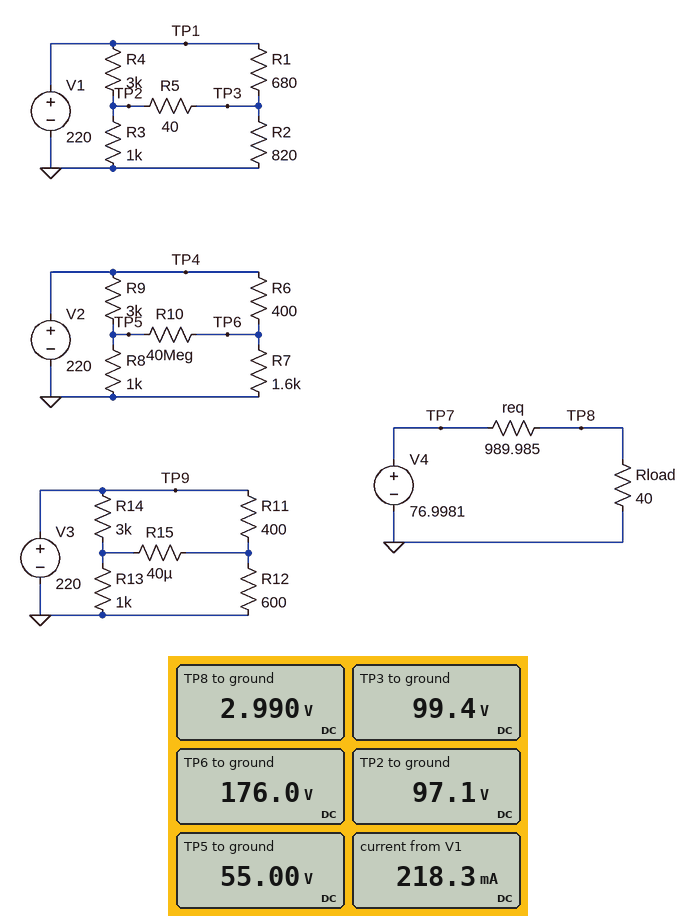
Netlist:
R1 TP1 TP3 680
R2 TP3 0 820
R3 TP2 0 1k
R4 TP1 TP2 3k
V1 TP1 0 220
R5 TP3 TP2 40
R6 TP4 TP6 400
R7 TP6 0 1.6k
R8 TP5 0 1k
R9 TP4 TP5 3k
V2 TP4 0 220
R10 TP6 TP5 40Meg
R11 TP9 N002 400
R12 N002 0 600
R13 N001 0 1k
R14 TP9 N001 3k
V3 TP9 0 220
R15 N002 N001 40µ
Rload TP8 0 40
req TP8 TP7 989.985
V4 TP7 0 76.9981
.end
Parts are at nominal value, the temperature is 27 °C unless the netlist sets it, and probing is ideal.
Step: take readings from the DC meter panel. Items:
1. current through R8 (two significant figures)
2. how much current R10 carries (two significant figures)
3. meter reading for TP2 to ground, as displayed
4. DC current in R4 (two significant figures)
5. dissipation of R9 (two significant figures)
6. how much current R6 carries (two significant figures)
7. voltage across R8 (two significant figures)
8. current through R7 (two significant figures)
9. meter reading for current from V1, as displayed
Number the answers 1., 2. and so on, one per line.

1. 55 mA
2. 3.0 µA
3. 97.1 V
4. 41 mA
5. 9.1 W
6. 110 mA
7. 55 V
8. 110 mA
9. 218.3 mA
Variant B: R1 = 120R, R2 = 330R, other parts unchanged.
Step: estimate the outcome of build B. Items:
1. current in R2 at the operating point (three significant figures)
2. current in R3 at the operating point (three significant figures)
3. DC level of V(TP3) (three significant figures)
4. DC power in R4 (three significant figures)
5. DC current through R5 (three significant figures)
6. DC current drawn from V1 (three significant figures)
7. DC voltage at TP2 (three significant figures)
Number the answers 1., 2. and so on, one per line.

1. 457 mA
2. 146 mA
3. 151 V
4. 1.83 W
5. 121 mA
6. 602 mA
7. 146 V
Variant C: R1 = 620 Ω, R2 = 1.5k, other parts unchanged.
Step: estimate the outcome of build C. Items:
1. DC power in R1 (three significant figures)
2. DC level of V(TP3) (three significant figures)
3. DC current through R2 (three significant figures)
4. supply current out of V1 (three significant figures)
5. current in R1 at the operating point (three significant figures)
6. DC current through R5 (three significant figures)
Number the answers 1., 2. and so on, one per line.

1. 16.2 W
2. 120 V
3. 79.8 mA
4. 196 mA
5. 162 mA
6. 81.9 mA
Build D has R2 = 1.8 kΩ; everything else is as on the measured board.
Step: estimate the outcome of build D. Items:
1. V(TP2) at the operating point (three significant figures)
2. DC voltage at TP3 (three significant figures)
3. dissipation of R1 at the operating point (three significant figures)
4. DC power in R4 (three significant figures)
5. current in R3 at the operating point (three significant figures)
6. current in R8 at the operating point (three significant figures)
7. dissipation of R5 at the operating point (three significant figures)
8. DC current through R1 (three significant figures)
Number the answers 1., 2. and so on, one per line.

1. 116 V
2. 119 V
3. 14.9 W
4. 3.59 W
5. 116 mA
6. 55.0 mA
7. 266 mW
8. 148 mA
